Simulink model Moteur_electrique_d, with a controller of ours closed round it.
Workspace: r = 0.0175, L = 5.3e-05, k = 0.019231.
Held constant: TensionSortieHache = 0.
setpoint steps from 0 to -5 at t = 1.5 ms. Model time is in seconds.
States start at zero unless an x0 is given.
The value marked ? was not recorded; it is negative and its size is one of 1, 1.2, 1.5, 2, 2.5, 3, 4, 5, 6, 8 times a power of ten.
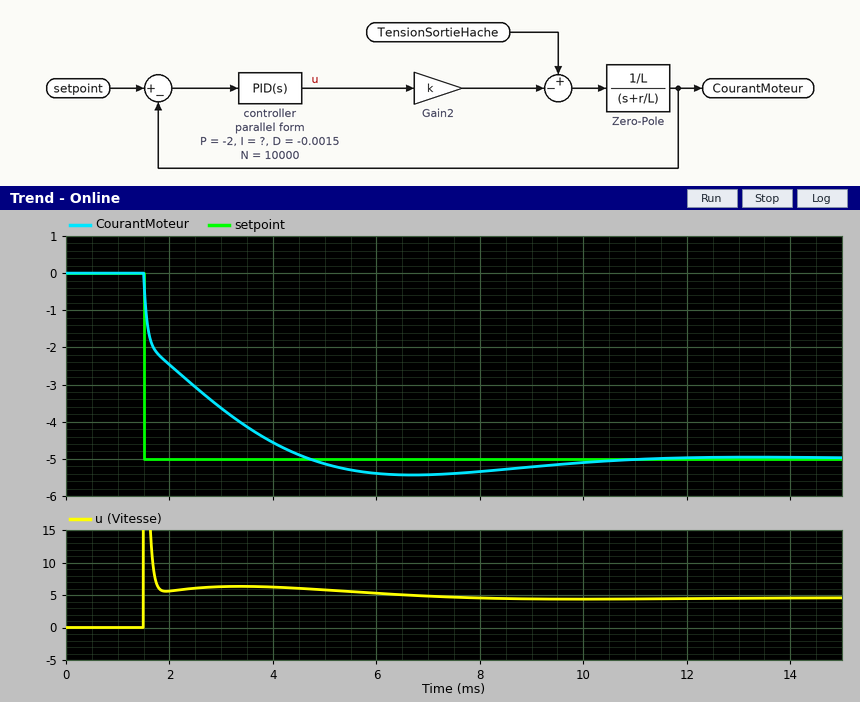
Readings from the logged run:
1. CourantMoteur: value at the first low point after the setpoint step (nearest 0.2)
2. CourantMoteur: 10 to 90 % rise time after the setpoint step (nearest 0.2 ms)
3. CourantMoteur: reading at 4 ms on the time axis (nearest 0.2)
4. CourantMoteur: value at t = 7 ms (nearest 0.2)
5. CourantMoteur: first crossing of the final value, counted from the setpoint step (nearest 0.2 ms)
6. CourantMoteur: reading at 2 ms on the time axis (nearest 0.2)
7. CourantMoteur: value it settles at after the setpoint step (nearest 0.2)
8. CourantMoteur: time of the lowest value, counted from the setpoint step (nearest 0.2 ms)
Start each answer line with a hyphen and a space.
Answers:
- -5.4
- 2.4 ms
- -4.6
- -5.4
- 3.2 ms
- -2.4
- -5.0
- 5.2 ms
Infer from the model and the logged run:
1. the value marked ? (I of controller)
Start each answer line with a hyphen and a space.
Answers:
- -1500
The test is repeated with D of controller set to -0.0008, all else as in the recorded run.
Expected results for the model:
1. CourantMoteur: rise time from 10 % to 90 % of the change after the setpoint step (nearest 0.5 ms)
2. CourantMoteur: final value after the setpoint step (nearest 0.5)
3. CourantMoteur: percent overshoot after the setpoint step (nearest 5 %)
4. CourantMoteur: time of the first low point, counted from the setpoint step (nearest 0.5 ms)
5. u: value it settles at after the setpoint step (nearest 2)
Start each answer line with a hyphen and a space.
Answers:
- 2.0 ms
- -5.0
- 10 %
- 4.5 ms
- 4
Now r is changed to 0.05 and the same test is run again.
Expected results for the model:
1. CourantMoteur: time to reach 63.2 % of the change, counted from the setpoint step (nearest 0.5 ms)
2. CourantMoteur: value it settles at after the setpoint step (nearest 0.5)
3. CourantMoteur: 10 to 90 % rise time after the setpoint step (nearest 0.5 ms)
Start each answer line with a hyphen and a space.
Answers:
- 2.0 ms
- -5.0
- 4.5 ms
